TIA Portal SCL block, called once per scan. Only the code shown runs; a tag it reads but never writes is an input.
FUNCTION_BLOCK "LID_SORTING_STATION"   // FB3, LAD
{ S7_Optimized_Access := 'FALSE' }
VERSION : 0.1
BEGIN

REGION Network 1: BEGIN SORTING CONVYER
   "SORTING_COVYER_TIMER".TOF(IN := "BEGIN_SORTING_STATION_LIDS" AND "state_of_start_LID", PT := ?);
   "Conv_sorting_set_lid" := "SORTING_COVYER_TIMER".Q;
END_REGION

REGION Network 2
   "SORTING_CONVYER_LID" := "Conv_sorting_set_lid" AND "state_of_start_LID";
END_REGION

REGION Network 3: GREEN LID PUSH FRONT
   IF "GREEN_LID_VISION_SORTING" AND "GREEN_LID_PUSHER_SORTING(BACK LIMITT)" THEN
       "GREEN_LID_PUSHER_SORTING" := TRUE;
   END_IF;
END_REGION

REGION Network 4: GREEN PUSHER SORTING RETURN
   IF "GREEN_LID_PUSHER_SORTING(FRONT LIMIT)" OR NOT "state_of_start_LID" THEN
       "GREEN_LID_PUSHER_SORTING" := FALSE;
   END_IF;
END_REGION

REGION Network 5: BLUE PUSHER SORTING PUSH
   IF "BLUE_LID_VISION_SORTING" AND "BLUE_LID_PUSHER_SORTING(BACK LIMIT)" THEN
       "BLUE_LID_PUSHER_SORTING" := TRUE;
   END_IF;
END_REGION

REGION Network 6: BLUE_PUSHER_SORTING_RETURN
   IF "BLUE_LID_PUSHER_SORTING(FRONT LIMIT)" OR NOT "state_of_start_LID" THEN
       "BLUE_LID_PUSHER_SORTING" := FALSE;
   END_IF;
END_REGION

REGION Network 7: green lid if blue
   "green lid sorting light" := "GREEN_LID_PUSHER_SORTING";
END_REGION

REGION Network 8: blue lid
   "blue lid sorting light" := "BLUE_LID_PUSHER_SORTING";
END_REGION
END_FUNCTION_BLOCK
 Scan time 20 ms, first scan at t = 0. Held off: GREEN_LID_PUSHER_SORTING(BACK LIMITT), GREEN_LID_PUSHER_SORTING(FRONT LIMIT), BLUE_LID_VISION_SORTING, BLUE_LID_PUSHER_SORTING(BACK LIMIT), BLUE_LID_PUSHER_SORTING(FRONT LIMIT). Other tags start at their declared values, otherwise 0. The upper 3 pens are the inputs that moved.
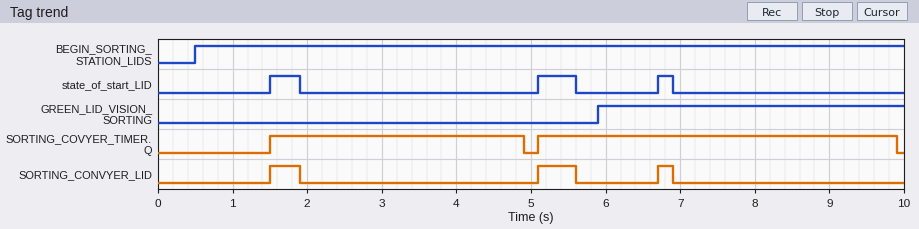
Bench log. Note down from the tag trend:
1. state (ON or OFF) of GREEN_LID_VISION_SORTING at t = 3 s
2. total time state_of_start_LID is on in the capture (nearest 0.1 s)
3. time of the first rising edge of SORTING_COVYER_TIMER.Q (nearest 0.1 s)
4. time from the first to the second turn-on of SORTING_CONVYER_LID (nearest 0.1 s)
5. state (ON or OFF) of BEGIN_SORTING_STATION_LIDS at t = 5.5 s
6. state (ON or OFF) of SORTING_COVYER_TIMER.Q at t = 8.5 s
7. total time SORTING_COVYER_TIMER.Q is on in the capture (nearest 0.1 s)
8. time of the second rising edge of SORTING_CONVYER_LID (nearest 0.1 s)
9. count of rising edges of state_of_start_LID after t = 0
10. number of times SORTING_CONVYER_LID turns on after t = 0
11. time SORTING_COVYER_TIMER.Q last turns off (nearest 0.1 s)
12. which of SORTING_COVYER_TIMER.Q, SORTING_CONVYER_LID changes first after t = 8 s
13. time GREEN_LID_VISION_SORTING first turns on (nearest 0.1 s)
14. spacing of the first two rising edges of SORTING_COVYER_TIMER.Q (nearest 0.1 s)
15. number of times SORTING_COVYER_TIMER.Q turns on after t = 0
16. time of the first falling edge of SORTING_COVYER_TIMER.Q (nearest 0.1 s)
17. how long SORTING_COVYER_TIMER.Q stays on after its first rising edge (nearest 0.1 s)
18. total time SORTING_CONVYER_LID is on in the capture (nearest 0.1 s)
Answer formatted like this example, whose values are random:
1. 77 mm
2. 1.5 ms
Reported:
1. OFF
2. 1.1 s
3. 1.5 s
4. 3.6 s
5. ON
6. ON
7. 8.2 s
8. 5.1 s
9. 3
10. 3
11. 9.9 s
12. SORTING_COVYER_TIMER.Q
13. 5.9 s
14. 3.6 s
15. 2
16. 4.9 s
17. 3.4 s
18. 1.1 s
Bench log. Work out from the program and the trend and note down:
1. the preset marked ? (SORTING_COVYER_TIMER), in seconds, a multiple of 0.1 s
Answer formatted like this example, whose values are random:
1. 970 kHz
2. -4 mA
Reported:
1. 3.0 s
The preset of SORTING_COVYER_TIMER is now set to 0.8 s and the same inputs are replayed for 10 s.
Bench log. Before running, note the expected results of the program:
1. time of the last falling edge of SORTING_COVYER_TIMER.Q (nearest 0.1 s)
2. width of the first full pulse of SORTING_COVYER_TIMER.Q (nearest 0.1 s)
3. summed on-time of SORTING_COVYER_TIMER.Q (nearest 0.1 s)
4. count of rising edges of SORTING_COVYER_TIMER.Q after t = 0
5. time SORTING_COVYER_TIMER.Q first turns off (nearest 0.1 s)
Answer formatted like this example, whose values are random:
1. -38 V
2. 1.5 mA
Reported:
1. 7.7 s
2. 1.2 s
3. 3.5 s
4. 3
5. 2.7 s
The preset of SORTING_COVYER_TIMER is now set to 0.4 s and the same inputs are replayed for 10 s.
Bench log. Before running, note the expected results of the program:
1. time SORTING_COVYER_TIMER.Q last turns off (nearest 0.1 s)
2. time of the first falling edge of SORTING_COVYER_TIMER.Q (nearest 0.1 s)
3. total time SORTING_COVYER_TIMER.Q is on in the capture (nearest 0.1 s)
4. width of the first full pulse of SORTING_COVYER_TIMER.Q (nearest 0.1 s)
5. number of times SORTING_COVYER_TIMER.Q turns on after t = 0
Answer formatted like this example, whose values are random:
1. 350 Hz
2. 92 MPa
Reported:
1. 7.3 s
2. 2.3 s
3. 2.3 s
4. 0.8 s
5. 3
